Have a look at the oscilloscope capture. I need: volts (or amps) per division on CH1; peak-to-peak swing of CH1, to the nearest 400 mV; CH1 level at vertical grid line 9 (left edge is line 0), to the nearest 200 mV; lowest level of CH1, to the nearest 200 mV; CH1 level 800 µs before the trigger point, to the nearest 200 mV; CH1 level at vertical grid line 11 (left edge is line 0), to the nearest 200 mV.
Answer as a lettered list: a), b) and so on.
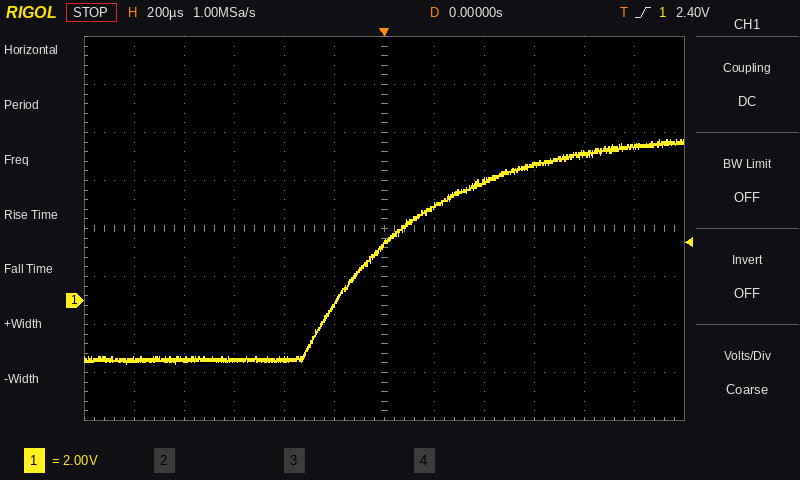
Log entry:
a) 2 V
b) 9.2 V
c) 5.6 V
d) -2.6 V
e) -2.4 V
f) 6.4 V
